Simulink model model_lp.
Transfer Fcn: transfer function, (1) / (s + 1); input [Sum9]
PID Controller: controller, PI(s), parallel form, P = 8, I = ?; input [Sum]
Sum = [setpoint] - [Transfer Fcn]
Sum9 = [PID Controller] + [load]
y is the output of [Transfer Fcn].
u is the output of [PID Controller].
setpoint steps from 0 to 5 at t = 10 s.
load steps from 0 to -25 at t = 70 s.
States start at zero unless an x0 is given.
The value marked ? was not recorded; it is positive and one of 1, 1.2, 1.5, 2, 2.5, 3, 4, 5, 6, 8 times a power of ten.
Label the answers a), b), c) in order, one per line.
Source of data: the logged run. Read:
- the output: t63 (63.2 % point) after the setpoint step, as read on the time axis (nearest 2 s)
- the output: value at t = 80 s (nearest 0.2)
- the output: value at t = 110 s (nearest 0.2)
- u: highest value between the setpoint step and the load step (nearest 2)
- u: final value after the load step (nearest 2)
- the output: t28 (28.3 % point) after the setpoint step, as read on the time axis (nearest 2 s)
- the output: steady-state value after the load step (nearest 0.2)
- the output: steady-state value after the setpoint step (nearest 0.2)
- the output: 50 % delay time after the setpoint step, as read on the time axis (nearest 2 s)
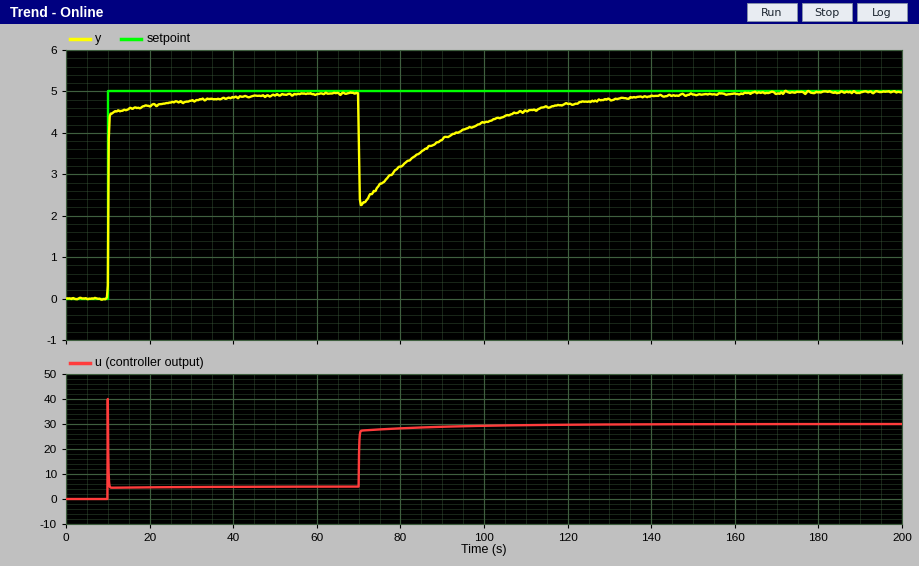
a) 10 s
b) 3.2
c) 4.6
d) 40
e) 30
f) 10 s
g) 5.0
h) 5.0
i) 10 s
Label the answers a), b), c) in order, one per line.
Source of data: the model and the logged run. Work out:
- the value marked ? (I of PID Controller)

a) 0.4
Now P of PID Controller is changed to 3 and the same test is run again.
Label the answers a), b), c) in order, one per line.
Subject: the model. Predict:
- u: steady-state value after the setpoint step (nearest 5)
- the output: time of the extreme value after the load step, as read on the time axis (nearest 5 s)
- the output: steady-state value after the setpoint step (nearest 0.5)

a) 5
b) 70 s
c) 5.0
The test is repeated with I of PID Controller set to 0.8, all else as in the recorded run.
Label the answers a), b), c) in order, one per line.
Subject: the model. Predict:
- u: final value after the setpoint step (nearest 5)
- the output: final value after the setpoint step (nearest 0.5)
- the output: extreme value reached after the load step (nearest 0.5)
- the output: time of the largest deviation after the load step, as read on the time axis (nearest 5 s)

a) 5
b) 5.0
c) 2.5
d) 70 s
